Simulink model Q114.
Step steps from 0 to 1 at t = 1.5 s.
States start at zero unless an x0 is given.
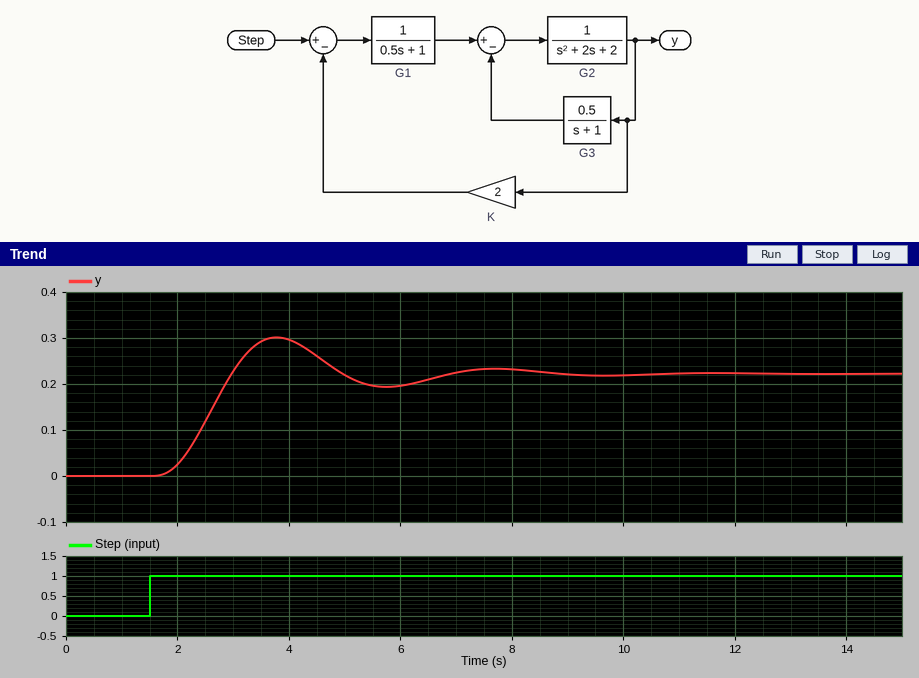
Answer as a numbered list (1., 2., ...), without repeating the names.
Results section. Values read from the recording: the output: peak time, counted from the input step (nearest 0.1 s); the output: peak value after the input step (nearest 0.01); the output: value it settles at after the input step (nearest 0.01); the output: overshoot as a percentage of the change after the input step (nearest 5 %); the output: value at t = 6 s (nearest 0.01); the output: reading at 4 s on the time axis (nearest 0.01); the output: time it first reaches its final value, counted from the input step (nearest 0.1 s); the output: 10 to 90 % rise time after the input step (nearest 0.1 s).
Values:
1. 2.3 s
2. 0.30
3. 0.22
4. 35 %
5. 0.20
6. 0.30
7. 1.5 s
8. 0.9 s
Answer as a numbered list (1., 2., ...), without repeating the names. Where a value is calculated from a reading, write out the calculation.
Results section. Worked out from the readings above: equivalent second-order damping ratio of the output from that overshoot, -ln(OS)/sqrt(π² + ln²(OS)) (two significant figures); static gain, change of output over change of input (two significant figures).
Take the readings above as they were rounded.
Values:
1. ln(0.35) = -1.050; 1.050 / sqrt(9.870 + 1.102) = 0.32
2. (0.22 - 0) / (1 - 0) = 0.22
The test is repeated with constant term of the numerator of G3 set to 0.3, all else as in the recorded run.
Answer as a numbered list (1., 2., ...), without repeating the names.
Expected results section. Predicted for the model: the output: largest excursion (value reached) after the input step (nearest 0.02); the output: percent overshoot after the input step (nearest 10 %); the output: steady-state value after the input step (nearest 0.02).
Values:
1. 0.30
2. 30 %
3. 0.24
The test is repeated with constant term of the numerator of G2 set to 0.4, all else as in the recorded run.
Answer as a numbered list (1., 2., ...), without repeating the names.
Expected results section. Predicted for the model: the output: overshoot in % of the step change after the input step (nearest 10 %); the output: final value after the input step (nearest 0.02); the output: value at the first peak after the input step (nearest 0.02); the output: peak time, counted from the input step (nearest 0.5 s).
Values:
1. 20 %
2. 0.14
3. 0.16
4. 3.0 s
